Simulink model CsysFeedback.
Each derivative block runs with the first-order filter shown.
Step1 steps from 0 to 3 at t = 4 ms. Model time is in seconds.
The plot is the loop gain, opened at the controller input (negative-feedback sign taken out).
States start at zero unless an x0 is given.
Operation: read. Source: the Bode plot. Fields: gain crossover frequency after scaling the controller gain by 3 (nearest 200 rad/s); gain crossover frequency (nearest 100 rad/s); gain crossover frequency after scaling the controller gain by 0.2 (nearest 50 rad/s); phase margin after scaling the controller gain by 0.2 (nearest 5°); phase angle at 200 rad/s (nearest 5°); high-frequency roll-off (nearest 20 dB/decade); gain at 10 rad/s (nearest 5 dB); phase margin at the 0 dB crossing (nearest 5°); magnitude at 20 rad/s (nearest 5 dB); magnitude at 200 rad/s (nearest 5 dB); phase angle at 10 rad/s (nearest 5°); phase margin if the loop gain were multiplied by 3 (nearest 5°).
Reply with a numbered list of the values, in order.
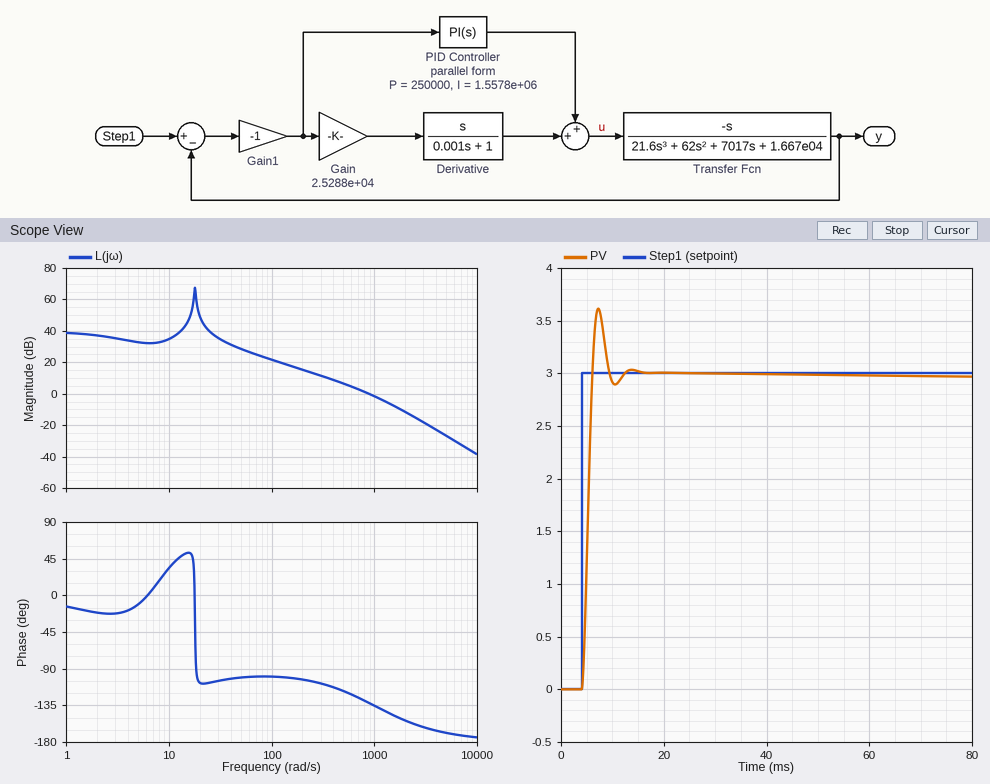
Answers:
1. 1800 rad/s
2. 900 rad/s
3. 250 rad/s
4. 75°
5. -105°
6. -40 dB/decade
7. 35 dB
8. 50°
9. 50 dB
10. 15 dB
11. 35°
12. 30°
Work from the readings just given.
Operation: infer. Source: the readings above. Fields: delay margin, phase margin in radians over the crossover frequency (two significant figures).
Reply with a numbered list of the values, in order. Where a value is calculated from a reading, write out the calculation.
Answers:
1. 50 × π / 180 / 900 = 0.00097 s
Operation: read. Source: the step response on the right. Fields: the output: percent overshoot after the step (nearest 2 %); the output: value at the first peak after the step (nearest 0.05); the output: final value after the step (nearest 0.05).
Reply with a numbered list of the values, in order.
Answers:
1. 22 %
2. 3.60
3. 2.95
